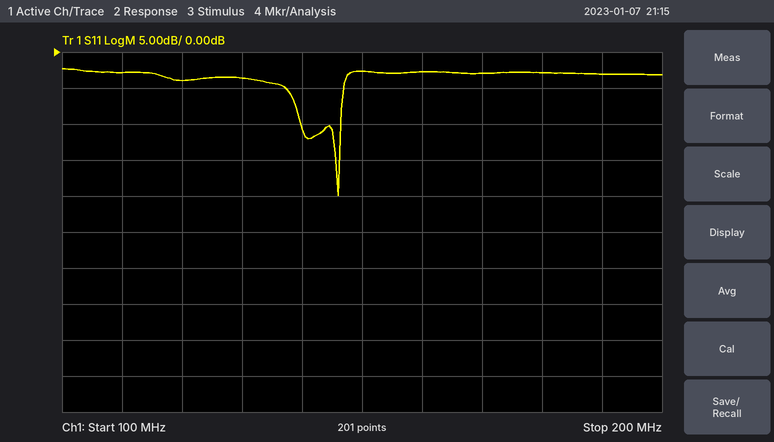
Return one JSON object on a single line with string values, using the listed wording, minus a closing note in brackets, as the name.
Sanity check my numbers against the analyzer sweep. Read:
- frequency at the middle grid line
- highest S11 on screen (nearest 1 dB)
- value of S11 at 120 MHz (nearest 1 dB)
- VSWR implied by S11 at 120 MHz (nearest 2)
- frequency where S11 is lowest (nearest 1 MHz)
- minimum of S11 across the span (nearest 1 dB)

{"frequency at the middle grid line": "150 MHz", "highest S11 on screen": "-2 dB", "value of S11 at 120 MHz": "-4 dB", "VSWR implied by S11 at 120 MHz": "4", "frequency where S11 is lowest": "146 MHz", "minimum of S11 across the span": "-20 dB"}
